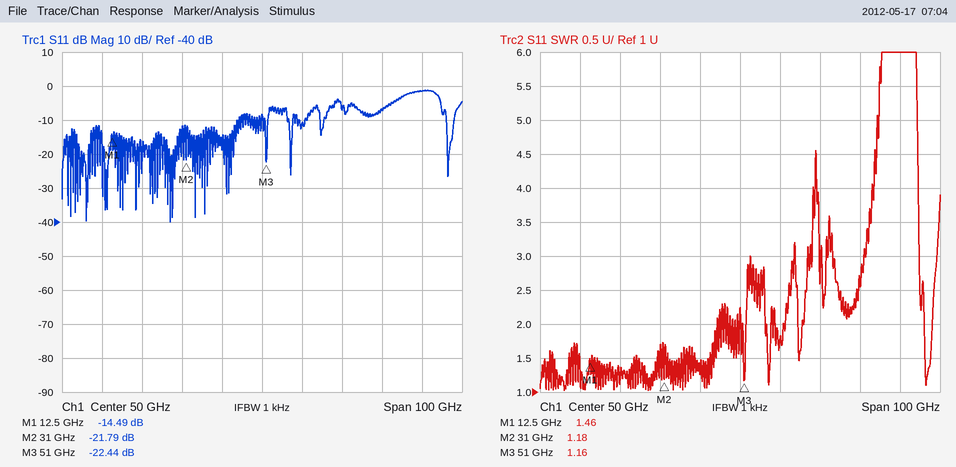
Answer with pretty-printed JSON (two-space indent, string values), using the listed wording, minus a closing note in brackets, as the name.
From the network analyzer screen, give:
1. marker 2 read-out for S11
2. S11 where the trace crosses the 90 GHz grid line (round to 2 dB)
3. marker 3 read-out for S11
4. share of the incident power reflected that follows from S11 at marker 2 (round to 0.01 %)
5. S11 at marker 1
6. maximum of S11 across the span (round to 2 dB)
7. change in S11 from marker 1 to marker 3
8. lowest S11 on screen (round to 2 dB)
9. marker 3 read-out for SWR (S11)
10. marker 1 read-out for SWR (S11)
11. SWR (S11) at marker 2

{
  "marker 2 read-out for S11": "-21.79 dB",
  "S11 where the trace crosses the 90 GHz grid line": "-2 dB",
  "marker 3 read-out for S11": "-22.44 dB",
  "share of the incident power reflected that follows from S11 at marker 2": "0.66 %",
  "S11 at marker 1": "-14.49 dB",
  "maximum of S11 across the span": "-2 dB",
  "change in S11 from marker 1 to marker 3": "-7.95 dB",
  "lowest S11 on screen": "-40 dB",
  "marker 3 read-out for SWR": "1.16",
  "marker 1 read-out for SWR": "1.46",
  "SWR (S11) at marker 2": "1.18"
}
